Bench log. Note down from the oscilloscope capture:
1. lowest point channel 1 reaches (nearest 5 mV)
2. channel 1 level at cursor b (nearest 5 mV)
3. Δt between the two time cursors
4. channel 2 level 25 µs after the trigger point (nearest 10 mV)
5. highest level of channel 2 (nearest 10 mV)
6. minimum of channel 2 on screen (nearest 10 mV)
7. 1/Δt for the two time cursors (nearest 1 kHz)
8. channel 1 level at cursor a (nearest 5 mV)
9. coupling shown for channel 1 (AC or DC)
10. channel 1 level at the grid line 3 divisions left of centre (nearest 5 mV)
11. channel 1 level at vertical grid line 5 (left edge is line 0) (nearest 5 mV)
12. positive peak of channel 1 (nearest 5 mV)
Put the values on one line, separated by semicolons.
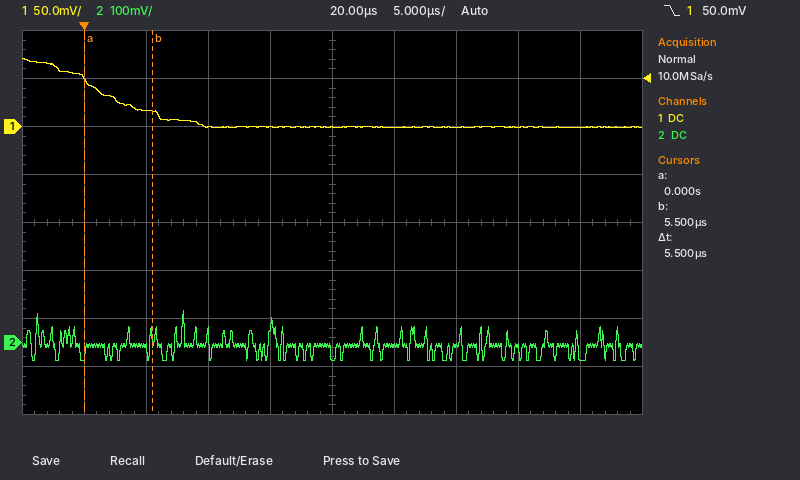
0 mV; 15 mV; 5.5 µs; -10 mV; 70 mV; -40 mV; 182 kHz; 50 mV; DC; 15 mV; 0 mV; 70 mV
